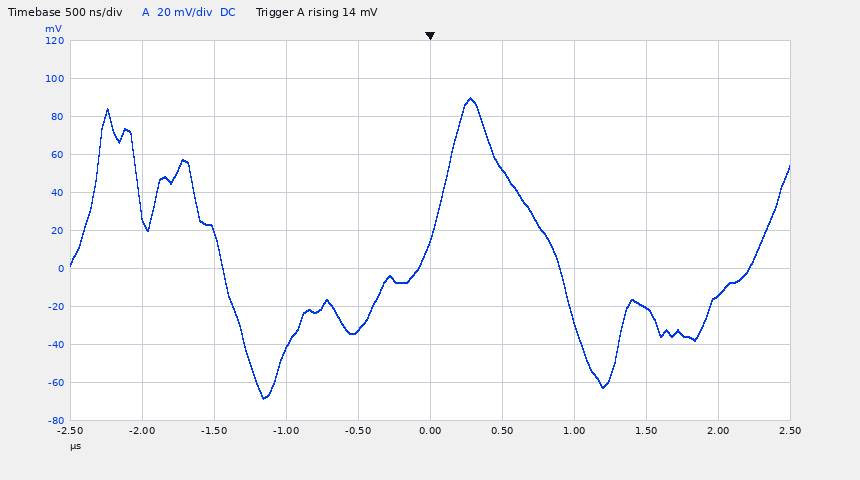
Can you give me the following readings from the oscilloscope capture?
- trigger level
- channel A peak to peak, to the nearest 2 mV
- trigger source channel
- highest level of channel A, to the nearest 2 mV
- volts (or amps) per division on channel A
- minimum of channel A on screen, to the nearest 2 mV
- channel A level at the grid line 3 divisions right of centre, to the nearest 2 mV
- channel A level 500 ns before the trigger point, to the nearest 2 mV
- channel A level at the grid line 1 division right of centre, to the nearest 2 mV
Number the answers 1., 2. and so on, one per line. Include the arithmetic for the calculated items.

1. 14 mV
2. 90 mV − (-68 mV) = 158 mV
3. channel A
4. 90 mV
5. 20 mV
6. -68 mV
7. -20 mV
8. -32 mV
9. 52 mV
